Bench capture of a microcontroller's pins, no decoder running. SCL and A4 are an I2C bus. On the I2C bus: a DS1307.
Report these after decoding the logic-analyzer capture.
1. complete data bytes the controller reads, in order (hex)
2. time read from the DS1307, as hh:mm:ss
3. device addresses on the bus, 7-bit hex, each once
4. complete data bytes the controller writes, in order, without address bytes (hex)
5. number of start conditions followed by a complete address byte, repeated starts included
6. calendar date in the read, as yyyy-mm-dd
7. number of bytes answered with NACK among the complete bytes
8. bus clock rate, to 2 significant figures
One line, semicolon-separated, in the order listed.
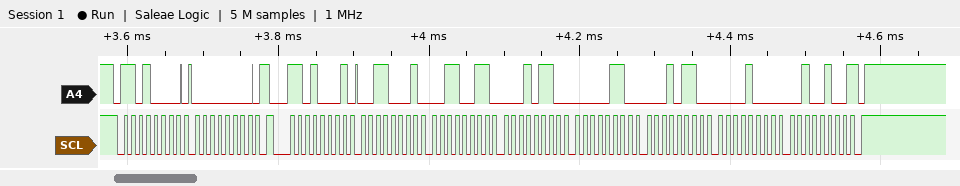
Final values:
31 33 16 06 16 08 24; 16:33:31; 0x68; 00; 2; 2024-08-16; 1; 100 kHz
